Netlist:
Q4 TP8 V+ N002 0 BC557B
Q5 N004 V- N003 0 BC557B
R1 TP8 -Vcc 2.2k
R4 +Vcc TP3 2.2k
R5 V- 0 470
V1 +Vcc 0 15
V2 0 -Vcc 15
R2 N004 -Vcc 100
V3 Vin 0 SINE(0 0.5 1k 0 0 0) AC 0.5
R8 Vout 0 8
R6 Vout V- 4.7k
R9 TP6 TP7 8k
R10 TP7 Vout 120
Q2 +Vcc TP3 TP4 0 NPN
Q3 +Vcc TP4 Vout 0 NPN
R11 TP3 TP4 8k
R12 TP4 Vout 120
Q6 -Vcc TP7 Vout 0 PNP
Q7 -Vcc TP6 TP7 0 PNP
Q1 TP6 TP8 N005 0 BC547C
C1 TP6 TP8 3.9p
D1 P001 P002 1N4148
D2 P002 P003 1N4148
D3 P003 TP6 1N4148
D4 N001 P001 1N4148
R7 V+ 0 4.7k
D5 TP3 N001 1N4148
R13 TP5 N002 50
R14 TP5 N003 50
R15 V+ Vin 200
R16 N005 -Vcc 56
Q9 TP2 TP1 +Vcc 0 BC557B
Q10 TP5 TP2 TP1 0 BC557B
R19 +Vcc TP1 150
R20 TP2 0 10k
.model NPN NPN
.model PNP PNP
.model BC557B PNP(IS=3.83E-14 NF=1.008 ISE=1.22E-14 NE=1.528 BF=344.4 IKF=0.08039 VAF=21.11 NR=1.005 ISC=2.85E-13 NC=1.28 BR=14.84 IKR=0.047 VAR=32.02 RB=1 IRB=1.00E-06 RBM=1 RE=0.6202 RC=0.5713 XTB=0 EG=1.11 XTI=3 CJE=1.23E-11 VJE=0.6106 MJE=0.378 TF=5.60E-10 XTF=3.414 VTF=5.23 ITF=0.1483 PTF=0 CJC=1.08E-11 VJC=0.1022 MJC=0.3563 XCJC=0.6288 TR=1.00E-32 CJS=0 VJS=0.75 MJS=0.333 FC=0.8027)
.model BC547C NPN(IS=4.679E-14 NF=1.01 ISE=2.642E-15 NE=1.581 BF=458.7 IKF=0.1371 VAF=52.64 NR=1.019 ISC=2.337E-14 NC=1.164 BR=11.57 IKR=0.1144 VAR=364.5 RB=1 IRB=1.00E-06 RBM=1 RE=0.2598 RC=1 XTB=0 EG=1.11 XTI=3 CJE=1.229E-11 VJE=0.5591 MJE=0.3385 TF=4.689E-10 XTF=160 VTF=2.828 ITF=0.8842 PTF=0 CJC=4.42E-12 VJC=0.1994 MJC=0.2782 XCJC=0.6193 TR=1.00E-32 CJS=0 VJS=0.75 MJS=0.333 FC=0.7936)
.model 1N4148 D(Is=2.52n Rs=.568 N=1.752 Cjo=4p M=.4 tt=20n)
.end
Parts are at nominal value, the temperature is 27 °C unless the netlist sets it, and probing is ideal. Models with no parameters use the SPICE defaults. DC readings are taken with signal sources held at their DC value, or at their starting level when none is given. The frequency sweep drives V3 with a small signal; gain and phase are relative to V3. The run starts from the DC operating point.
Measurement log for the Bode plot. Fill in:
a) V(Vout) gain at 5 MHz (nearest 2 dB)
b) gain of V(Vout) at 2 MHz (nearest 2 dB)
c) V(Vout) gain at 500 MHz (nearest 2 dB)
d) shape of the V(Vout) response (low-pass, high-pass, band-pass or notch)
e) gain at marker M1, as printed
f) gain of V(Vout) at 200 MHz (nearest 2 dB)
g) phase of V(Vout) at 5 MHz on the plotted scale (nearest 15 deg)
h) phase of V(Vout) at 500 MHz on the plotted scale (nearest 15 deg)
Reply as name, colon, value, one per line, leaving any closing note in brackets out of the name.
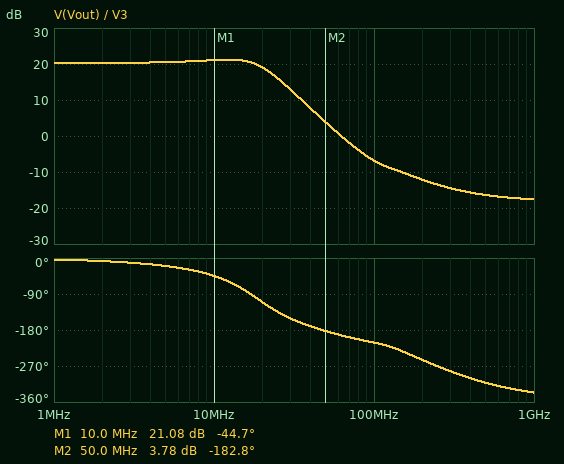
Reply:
V(Vout) gain at 5 MHz: 20 dB
gain of V(Vout) at 2 MHz: 20 dB
V(Vout) gain at 500 MHz: -16 dB
shape of the V(Vout) response: low-pass
gain at marker M1, as printed: 21.08 dB
gain of V(Vout) at 200 MHz: -12 dB
phase of V(Vout) at 5 MHz on the plotted scale: -15 deg
phase of V(Vout) at 500 MHz on the plotted scale: -315 deg
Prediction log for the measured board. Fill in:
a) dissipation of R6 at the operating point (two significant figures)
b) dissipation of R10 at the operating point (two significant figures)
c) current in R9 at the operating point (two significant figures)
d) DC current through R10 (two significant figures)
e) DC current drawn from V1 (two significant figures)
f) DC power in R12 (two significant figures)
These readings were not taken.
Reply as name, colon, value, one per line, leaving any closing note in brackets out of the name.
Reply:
dissipation of R6 at the operating point: 1.0 mW
dissipation of R10 at the operating point: 7.1 mW
current in R9 at the operating point: 100 µA
DC current through R10: 7.7 mA
DC current drawn from V1: 22 mA
DC power in R12: 5.4 mW
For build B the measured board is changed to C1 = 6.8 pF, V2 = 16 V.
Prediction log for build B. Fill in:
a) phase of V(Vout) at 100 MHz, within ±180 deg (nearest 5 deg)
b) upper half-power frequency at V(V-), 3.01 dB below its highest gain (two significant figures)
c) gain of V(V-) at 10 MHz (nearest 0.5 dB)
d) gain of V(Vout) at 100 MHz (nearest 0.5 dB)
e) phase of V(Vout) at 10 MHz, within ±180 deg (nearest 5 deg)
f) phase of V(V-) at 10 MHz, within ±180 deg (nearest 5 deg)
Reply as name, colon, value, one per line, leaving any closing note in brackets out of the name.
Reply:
phase of V(Vout) at 100 MHz, within ±180 deg: 145 deg
upper half-power frequency at V(V-), 3.01 dB below its highest gain: 11 MHz
gain of V(V-) at 10 MHz: -2.5 dB
gain of V(Vout) at 100 MHz: -10.0 dB
phase of V(Vout) at 10 MHz, within ±180 deg: -65 deg
phase of V(V-) at 10 MHz, within ±180 deg: -70 deg
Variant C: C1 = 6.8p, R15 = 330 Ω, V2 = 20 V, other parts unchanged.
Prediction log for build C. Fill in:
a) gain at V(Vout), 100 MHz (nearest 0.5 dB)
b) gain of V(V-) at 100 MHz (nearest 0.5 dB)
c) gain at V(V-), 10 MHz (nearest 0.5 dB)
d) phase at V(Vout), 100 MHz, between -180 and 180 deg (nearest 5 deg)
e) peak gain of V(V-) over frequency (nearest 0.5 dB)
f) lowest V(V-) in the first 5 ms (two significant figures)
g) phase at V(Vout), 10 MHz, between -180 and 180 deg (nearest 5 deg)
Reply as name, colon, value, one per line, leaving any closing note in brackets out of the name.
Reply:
gain at V(Vout), 100 MHz: -12.0 dB
gain of V(V-) at 100 MHz: -8.5 dB
gain at V(V-), 10 MHz: -2.5 dB
phase at V(Vout), 100 MHz, between -180 and 180 deg: 140 deg
peak gain of V(V-) over frequency: -1.0 dB
lowest V(V-) in the first 5 ms: -670 mV
phase at V(Vout), 10 MHz, between -180 and 180 deg: -70 deg
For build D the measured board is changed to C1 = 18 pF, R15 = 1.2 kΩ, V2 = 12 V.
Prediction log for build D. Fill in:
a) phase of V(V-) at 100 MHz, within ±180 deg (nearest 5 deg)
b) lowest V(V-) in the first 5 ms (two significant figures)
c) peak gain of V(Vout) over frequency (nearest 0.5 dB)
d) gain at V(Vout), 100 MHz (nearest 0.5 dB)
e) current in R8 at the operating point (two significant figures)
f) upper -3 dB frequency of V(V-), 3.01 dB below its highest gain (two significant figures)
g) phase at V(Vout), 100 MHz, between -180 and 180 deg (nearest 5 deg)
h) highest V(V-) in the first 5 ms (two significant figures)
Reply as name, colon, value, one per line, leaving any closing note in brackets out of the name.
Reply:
phase of V(V-) at 100 MHz, within ±180 deg: -35 deg
lowest V(V-) in the first 5 ms: -600 mV
peak gain of V(Vout) over frequency: 18.5 dB
gain at V(Vout), 100 MHz: -25.0 dB
current in R8 at the operating point: 300 mA
upper -3 dB frequency of V(V-), 3.01 dB below its highest gain: 5.3 MHz
phase at V(Vout), 100 MHz, between -180 and 180 deg: 105 deg
highest V(V-) in the first 5 ms: 170 mV
